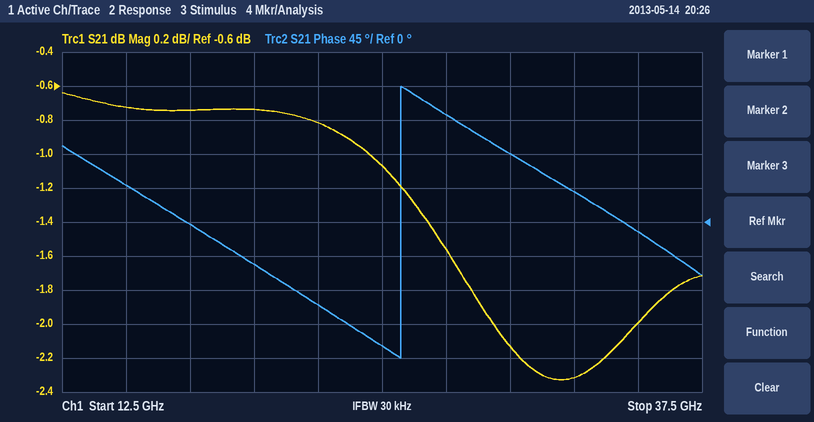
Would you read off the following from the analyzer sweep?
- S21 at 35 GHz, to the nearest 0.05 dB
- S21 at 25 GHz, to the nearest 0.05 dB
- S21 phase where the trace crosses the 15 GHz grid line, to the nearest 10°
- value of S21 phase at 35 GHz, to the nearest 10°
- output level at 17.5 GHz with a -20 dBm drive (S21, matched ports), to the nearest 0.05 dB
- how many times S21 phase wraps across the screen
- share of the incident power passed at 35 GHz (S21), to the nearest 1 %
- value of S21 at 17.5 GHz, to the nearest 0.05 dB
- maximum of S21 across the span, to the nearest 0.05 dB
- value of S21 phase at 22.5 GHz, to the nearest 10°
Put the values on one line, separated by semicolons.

-2.00 dB; -1.05 dB; 50°; -10°; -20.75 dBm; 1; 63 %; -0.75 dB; -0.65 dB; -110°
